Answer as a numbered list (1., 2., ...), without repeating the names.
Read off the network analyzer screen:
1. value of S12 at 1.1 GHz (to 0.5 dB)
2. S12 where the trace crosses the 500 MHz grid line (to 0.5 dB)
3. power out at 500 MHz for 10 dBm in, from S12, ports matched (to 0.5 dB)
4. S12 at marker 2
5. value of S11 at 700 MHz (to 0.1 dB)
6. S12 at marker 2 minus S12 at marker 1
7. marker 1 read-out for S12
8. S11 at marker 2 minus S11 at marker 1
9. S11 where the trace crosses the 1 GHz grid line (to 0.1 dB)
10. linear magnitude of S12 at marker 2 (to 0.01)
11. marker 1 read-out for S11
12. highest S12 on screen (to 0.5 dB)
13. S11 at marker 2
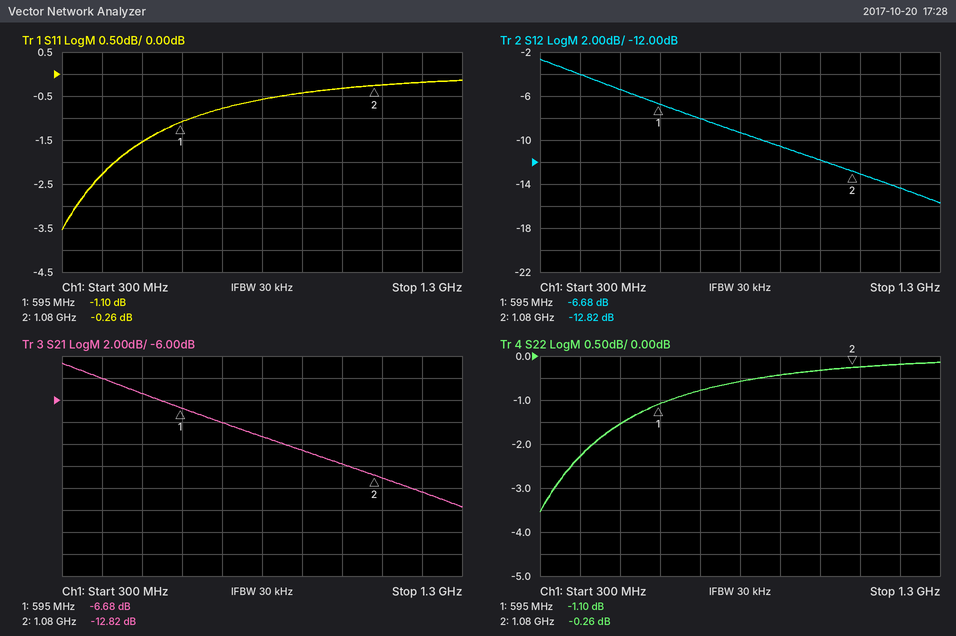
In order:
1. -13.0 dB
2. -5.5 dB
3. 4.5 dBm
4. -12.82 dB
5. -0.8 dB
6. -6.14 dB
7. -6.68 dB
8. 0.84 dB
9. -0.3 dB
10. 0.23
11. -1.10 dB
12. -2.5 dB
13. -0.26 dB
